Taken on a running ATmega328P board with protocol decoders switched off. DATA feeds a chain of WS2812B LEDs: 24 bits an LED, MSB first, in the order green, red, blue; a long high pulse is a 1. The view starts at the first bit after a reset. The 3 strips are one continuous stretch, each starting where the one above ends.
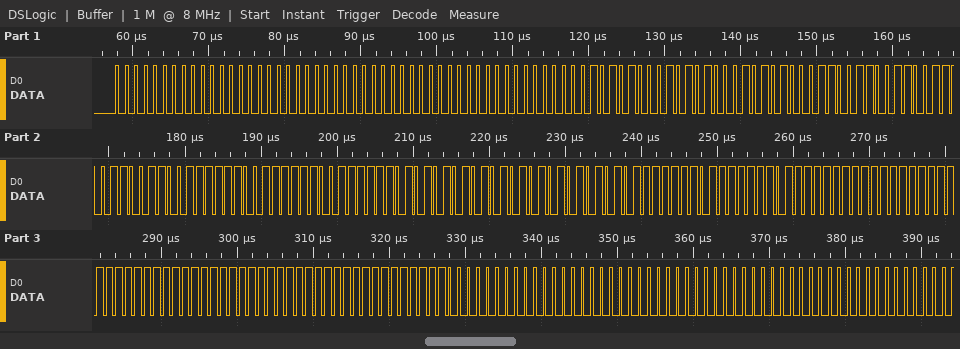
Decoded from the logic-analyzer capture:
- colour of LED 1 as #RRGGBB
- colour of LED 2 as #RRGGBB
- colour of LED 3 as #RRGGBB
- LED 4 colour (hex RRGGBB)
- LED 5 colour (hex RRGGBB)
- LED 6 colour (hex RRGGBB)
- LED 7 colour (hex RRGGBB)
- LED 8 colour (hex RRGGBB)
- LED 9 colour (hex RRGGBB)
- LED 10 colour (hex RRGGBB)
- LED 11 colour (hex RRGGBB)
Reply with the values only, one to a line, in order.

#000000
#000000
#2A2A2A
#333333
#3F3F3F
#555555
#7F7F7F
#FFFFFF
#FFFFFF
#000000
#000000
